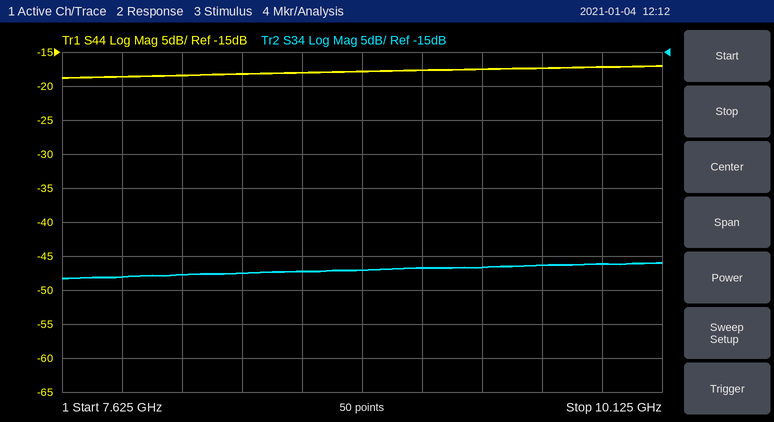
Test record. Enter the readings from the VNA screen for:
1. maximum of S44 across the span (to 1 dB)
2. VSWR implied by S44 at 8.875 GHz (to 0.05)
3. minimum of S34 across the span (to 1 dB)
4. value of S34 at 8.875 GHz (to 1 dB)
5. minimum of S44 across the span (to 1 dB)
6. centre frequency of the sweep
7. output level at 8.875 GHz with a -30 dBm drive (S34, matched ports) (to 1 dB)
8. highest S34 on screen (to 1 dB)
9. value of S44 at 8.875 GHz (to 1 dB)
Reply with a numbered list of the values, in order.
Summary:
1. -17 dB
2. 1.30
3. -48 dB
4. -47 dB
5. -19 dB
6. 8.875 GHz
7. -77 dBm
8. -46 dB
9. -18 dB
